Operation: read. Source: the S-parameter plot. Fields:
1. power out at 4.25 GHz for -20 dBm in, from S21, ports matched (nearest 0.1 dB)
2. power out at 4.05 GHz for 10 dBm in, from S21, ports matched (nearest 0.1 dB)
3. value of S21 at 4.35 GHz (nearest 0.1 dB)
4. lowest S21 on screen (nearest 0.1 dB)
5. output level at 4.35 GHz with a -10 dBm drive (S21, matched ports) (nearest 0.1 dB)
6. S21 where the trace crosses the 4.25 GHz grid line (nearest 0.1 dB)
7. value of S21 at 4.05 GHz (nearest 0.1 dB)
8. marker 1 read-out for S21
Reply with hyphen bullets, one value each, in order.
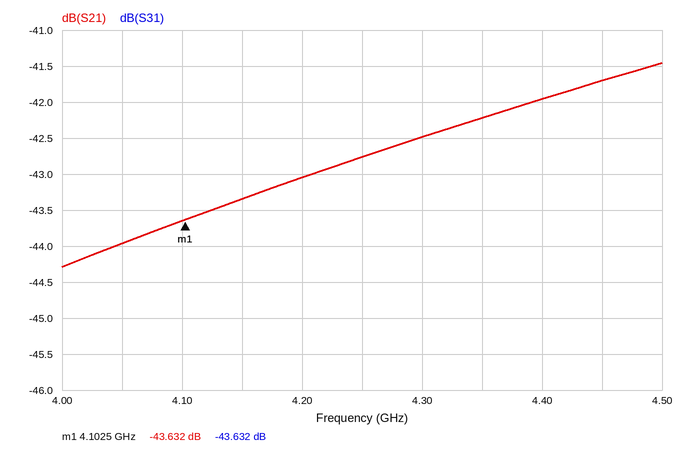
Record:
- -62.8 dBm
- -34.0 dBm
- -42.2 dB
- -44.3 dB
- -52.2 dBm
- -42.8 dB
- -44.0 dB
- -43.632 dB
